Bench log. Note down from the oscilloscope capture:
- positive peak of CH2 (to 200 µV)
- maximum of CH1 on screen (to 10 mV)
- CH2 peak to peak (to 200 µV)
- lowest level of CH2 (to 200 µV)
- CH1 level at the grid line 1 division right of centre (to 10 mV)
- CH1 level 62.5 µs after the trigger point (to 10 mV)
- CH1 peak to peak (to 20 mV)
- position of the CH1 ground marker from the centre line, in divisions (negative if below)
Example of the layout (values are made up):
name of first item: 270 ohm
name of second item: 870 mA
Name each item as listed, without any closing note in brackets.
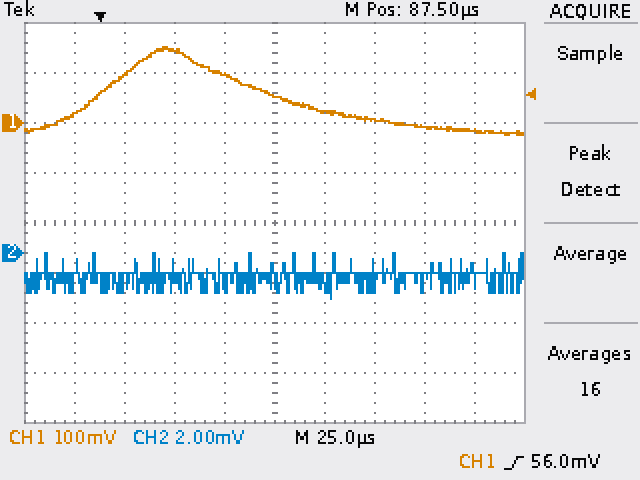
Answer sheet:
positive peak of CH2: 0.0 mV
maximum of CH1 on screen: 150 mV
CH2 peak to peak: 1.8 mV
lowest level of CH2: -1.8 mV
CH1 level at the grid line 1 division right of centre: 20 mV
CH1 level 62.5 µs after the trigger point: 100 mV
CH1 peak to peak: 180 mV
position of the CH1 ground marker from the centre line, in divisions: +2.0 div
